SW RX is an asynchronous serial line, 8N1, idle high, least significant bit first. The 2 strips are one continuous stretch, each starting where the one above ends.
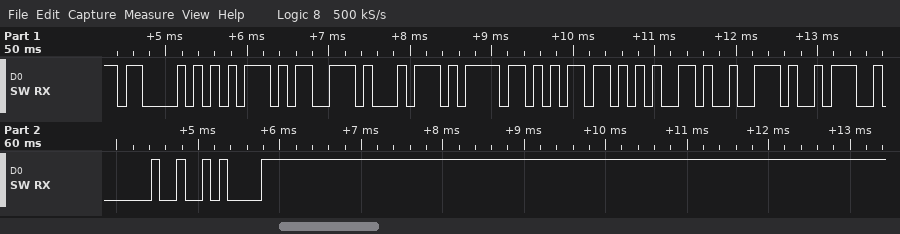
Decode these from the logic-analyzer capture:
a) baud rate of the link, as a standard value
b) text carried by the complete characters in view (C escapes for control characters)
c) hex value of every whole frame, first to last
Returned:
9600 baud
"Customer: \n"
43 75 73 74 6F 6D 65 72 3A 20 0A
